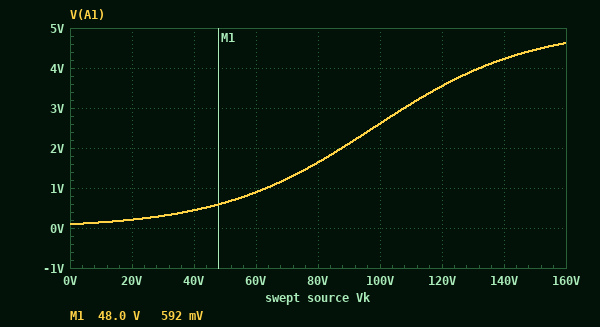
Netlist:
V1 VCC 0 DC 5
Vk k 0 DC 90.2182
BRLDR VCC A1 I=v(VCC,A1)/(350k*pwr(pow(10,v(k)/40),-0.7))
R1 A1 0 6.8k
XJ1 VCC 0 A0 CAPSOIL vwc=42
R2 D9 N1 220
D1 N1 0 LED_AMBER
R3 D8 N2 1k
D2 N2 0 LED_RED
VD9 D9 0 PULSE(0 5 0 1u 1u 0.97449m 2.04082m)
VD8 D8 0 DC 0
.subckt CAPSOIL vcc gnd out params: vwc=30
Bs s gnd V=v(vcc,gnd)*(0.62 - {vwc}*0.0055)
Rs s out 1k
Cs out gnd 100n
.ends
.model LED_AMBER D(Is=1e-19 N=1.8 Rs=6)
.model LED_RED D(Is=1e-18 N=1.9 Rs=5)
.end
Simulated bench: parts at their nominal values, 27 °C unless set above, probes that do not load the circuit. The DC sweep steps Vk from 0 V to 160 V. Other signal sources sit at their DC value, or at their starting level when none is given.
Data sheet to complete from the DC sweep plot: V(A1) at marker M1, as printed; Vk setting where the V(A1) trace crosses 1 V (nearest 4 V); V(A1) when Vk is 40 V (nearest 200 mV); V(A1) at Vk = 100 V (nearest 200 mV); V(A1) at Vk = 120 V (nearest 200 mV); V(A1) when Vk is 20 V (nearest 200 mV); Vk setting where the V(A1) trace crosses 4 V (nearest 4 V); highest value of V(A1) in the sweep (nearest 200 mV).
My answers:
592 mV
64 V
400 mV
2.6 V
3.6 V
200 mV
132 V
4.6 V
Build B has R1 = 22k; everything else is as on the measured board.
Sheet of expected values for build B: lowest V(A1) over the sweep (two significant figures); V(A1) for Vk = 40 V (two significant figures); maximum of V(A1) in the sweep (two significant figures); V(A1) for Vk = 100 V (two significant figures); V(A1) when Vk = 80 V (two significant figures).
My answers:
300 mV
1.2 V
4.9 V
3.9 V
3.1 V
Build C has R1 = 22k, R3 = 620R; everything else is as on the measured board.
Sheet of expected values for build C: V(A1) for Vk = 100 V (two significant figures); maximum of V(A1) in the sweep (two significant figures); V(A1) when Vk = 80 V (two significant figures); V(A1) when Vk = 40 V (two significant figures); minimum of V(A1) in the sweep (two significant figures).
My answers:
3.9 V
4.9 V
3.1 V
1.2 V
300 mV
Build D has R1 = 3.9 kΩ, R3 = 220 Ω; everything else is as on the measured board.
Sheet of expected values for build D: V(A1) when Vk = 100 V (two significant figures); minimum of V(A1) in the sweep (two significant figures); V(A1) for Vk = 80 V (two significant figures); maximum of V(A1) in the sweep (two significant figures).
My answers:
1.9 V
55 mV
1.1 V
4.4 V
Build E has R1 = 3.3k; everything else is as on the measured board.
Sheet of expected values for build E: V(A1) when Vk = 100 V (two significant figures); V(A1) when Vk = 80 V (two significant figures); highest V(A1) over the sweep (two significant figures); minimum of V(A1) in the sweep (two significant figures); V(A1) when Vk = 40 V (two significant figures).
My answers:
1.7 V
960 mV
4.3 V
47 mV
230 mV
